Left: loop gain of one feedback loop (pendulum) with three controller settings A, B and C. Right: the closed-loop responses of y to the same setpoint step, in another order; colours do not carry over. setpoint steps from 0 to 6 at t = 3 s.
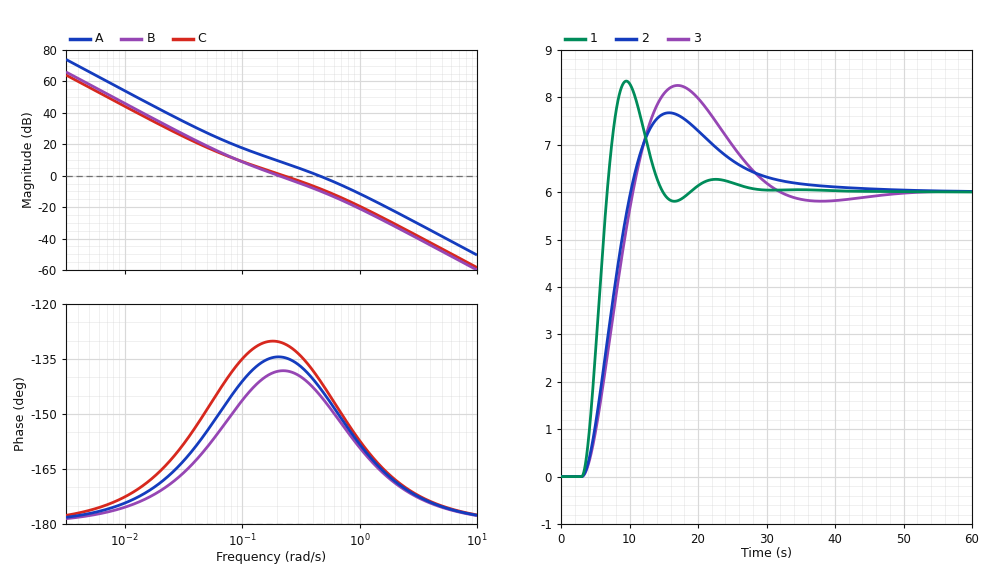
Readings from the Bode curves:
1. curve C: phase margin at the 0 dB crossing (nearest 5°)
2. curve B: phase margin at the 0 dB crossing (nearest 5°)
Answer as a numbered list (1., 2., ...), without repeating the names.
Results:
1. 50°
2. 40°
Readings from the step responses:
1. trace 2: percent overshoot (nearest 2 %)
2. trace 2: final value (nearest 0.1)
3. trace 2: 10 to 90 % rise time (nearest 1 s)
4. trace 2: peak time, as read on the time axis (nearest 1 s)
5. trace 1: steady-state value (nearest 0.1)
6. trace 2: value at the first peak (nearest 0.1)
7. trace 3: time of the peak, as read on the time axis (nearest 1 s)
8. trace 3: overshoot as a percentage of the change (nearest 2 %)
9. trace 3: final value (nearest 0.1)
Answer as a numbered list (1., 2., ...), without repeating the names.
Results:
1. 28 %
2. 6.0
3. 5 s
4. 16 s
5. 6.0
6. 7.7
7. 17 s
8. 38 %
9. 6.0
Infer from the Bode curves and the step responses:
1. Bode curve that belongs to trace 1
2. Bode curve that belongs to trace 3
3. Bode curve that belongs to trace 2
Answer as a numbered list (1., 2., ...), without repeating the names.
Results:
1. A
2. B
3. C
